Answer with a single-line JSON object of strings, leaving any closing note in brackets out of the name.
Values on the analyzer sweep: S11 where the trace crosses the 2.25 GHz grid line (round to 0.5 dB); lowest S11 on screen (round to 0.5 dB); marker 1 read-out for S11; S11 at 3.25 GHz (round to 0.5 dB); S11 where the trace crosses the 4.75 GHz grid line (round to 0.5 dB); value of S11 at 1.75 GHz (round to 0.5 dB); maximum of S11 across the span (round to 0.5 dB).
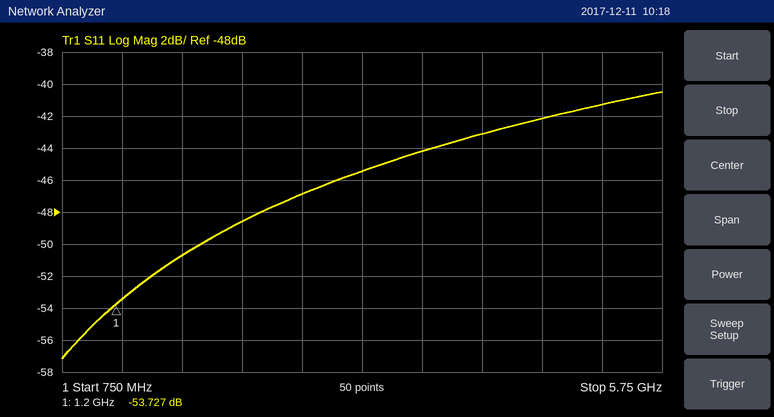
{"S11 where the trace crosses the 2.25 GHz grid line": "-48.5 dB", "lowest S11 on screen": "-57.0 dB", "marker 1 read-out for S11": "-53.727 dB", "S11 at 3.25 GHz": "-45.5 dB", "S11 where the trace crosses the 4.75 GHz grid line": "-42.0 dB", "value of S11 at 1.75 GHz": "-50.5 dB", "maximum of S11 across the span": "-40.5 dB"}
